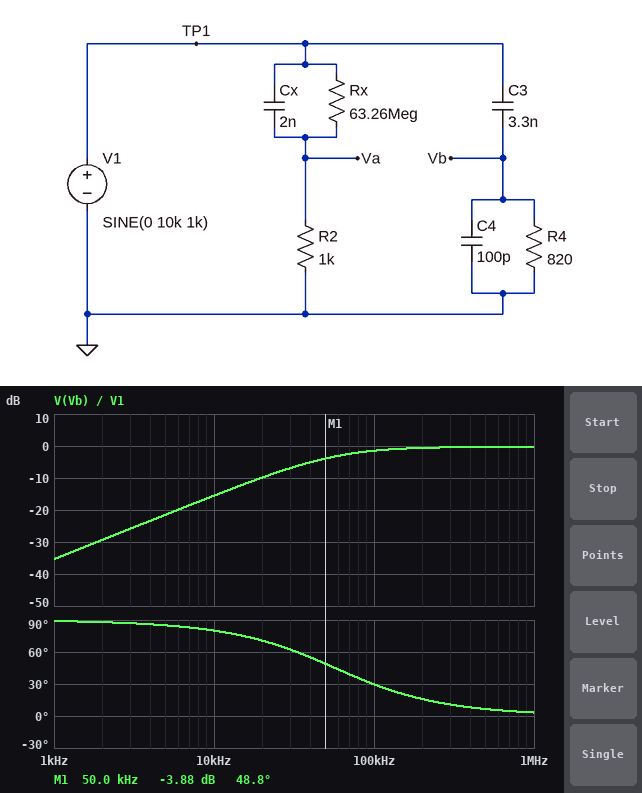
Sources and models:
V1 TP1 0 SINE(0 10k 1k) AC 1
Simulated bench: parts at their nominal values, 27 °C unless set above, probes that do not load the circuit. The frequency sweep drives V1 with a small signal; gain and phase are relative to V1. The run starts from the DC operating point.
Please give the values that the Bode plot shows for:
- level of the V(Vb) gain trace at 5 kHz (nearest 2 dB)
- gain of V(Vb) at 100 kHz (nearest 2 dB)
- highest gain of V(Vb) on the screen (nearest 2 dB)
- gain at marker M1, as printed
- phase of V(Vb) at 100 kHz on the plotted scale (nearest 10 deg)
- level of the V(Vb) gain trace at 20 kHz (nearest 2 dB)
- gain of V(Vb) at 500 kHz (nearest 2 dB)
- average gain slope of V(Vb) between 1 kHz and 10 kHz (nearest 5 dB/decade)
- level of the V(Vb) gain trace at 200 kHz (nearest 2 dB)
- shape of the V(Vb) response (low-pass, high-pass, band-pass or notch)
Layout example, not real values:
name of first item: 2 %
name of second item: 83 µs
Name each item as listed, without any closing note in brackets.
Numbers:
level of the V(Vb) gain trace at 5 kHz: -22 dB
gain of V(Vb) at 100 kHz: -2 dB
highest gain of V(Vb) on the screen: 0 dB
gain at marker M1, as printed: -3.88 dB
phase of V(Vb) at 100 kHz on the plotted scale: 30 deg
level of the V(Vb) gain trace at 20 kHz: -10 dB
gain of V(Vb) at 500 kHz: 0 dB
average gain slope of V(Vb) between 1 kHz and 10 kHz: 20 dB/decade
level of the V(Vb) gain trace at 200 kHz: 0 dB
shape of the V(Vb) response: high-pass
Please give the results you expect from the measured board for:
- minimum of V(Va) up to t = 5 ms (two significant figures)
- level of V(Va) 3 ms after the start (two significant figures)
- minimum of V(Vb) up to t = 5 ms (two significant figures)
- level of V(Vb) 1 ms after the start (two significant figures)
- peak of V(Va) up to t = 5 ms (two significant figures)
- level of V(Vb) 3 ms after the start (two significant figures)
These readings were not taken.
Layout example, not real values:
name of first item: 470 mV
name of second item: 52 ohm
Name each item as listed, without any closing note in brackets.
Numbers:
minimum of V(Va) up to t = 5 ms: -130 V
level of V(Va) 3 ms after the start: 130 V
minimum of V(Vb) up to t = 5 ms: -170 V
level of V(Vb) 1 ms after the start: 170 V
peak of V(Va) up to t = 5 ms: 130 V
level of V(Vb) 3 ms after the start: 170 V
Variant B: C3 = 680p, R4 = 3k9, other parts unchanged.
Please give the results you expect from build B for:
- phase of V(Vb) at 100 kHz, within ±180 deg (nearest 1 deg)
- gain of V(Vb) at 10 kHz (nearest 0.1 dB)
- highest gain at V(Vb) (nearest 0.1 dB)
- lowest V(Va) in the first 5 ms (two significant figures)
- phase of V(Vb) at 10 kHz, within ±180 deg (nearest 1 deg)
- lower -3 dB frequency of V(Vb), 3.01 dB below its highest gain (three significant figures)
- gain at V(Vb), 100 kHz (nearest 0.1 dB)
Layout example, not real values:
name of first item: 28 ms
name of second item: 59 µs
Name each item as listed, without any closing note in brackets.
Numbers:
phase of V(Vb) at 100 kHz, within ±180 deg: 28 deg
gain of V(Vb) at 10 kHz: -15.7 dB
highest gain at V(Vb): -1.2 dB
lowest V(Va) in the first 5 ms: -130 V
phase of V(Vb) at 10 kHz, within ±180 deg: 79 deg
lower -3 dB frequency of V(Vb), 3.01 dB below its highest gain: 52.3 kHz
gain at V(Vb), 100 kHz: -2.2 dB
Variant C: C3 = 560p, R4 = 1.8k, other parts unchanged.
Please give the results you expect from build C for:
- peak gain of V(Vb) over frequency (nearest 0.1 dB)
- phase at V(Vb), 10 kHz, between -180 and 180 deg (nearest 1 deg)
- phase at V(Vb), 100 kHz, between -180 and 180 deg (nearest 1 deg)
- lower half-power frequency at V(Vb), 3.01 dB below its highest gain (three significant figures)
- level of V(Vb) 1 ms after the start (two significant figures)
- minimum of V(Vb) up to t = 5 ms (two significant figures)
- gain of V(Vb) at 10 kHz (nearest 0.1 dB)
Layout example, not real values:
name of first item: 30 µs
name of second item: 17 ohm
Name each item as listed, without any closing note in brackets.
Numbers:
peak gain of V(Vb) over frequency: -1.4 dB
phase at V(Vb), 10 kHz, between -180 and 180 deg: 86 deg
phase at V(Vb), 100 kHz, between -180 and 180 deg: 53 deg
lower half-power frequency at V(Vb), 3.01 dB below its highest gain: 134 kHz
level of V(Vb) 1 ms after the start: 63 V
minimum of V(Vb) up to t = 5 ms: -63 V
gain of V(Vb) at 10 kHz: -24.0 dB
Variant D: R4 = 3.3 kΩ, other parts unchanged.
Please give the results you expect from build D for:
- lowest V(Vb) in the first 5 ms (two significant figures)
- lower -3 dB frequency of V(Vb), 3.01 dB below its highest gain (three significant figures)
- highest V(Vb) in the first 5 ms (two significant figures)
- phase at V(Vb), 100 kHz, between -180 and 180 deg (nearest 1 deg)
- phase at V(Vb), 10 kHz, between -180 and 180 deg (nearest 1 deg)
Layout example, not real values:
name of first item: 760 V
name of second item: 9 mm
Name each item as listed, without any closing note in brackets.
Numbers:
lowest V(Vb) in the first 5 ms: -680 V
lower -3 dB frequency of V(Vb), 3.01 dB below its highest gain: 14.2 kHz
highest V(Vb) in the first 5 ms: 680 V
phase at V(Vb), 100 kHz, between -180 and 180 deg: 8 deg
phase at V(Vb), 10 kHz, between -180 and 180 deg: 55 deg
